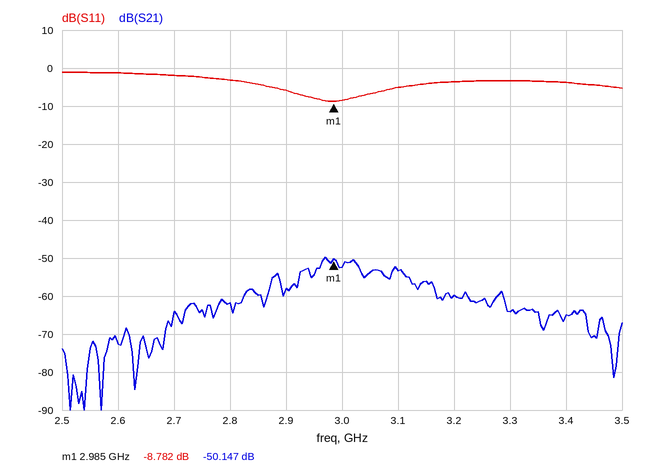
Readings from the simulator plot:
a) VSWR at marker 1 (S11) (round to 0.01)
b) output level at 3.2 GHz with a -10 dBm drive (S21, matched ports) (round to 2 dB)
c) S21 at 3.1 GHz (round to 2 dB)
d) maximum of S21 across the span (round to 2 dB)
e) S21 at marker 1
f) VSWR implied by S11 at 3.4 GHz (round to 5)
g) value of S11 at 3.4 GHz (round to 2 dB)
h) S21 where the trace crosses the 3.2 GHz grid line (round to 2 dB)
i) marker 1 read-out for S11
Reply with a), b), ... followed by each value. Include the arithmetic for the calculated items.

a) (1 + 0.3638)/(1 − 0.3638) ≈ 2.14
b) -10 dBm + (-60 dB) = -70 dBm
c) -54 dB
d) -50 dB
e) -50.147 dB
f) |Γ| = 10^(-4/20) = 0.6310; VSWR = (1 + 0.6310)/(1 − 0.6310) ≈ 4.42, so 5 to the nearest 5
g) -4 dB
h) -60 dB
i) -8.782 dB
